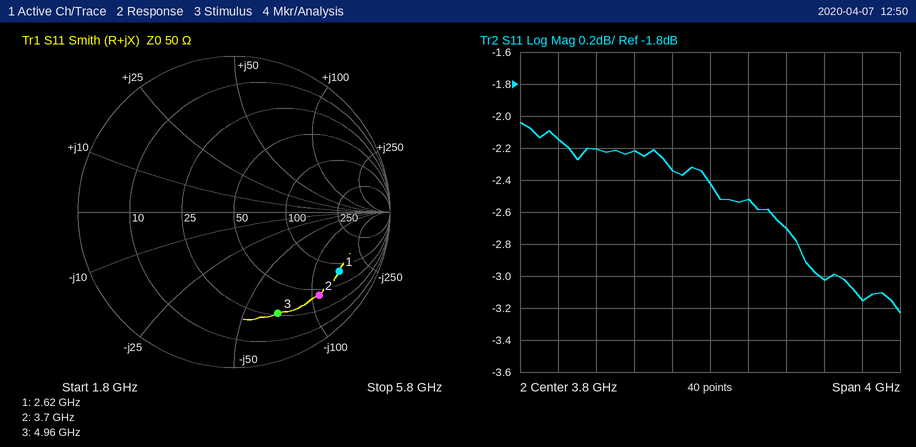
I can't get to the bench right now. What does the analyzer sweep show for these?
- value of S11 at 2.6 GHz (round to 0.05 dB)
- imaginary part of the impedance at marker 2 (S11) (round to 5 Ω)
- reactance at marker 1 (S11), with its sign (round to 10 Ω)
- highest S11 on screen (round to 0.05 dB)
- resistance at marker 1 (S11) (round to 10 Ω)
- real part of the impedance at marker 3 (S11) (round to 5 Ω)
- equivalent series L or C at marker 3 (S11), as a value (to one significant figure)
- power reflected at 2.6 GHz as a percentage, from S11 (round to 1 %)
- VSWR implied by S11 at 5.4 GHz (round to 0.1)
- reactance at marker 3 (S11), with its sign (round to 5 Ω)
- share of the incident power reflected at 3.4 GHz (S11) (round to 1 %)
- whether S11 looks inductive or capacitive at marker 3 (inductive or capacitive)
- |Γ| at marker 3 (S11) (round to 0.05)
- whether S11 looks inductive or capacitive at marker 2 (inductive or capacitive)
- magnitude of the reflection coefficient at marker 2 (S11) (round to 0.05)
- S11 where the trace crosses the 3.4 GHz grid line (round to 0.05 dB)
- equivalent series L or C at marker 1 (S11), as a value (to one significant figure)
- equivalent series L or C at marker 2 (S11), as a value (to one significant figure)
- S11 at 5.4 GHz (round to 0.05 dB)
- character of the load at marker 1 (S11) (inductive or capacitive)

-2.20 dB
-110 Ω
-150 Ω
-2.05 dB
80 Ω
25 Ω
500 fF
60 %
5.6
-70 Ω
58 %
capacitive
0.70
capacitive
0.75
-2.35 dB
400 fF
400 fF
-3.15 dB
capacitive
